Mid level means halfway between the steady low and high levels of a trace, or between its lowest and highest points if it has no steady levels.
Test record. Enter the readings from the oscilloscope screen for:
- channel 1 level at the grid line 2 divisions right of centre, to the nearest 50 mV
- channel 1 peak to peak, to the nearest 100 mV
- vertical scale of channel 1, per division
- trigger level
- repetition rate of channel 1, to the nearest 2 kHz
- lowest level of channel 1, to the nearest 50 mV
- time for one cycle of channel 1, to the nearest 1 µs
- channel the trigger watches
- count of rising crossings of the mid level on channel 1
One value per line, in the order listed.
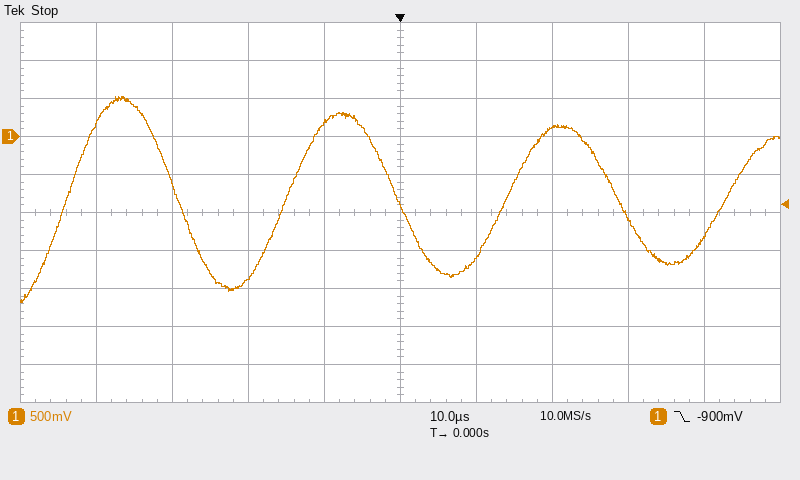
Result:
100 mV
2.70 V
500 mV
-900 mV
34 kHz
-2.20 V
29 µs
channel 1
4
